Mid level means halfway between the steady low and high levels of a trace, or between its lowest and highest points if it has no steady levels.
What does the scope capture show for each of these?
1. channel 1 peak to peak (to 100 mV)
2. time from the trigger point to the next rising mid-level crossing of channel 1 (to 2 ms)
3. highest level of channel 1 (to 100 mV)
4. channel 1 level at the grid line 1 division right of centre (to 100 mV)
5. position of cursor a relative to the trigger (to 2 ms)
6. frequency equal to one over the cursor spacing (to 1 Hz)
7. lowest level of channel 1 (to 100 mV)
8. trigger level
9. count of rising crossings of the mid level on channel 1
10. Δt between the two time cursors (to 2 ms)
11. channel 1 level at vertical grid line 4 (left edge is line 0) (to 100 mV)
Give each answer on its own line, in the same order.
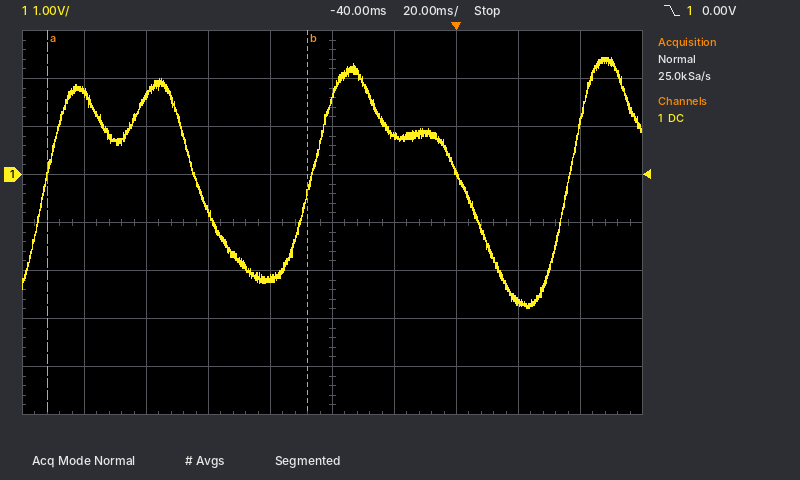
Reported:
5.2 V
36 ms
2.4 V
800 mV
-132 ms
12 Hz
-2.8 V
0.00 V
3
84 ms
-2.2 V
